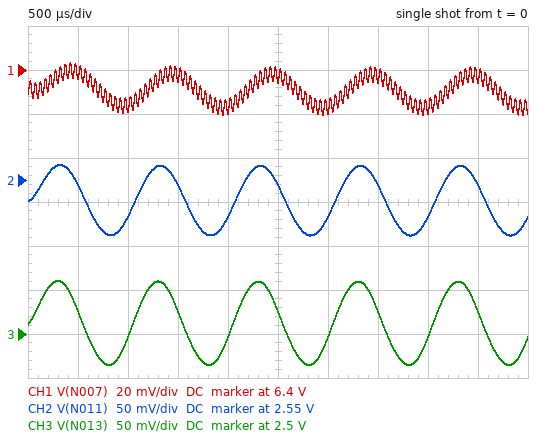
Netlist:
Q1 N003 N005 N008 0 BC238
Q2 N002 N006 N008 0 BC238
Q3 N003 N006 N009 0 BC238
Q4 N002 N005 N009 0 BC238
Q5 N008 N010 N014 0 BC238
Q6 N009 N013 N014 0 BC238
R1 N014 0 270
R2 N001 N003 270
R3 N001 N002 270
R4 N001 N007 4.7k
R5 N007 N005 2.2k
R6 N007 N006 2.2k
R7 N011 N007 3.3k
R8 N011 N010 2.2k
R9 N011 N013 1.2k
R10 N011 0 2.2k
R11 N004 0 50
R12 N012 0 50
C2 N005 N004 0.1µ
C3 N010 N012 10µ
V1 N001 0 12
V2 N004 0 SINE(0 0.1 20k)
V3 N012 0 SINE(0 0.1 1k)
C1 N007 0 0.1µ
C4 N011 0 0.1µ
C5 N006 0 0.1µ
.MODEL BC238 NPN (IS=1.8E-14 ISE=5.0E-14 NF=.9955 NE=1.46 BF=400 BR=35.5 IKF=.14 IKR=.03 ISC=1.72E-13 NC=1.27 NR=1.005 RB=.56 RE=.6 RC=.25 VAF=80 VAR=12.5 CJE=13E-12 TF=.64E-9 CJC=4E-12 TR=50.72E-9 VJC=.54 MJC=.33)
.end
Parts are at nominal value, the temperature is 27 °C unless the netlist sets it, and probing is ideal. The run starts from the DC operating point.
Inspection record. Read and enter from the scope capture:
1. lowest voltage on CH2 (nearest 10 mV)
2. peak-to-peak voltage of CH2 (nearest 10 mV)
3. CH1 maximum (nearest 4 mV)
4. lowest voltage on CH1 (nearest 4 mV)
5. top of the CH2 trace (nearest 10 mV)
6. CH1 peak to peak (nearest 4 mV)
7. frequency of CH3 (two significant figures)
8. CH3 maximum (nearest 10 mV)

2.49 V
80 mV
6.404 V
6.380 V
2.57 V
24 mV
1.0 kHz
2.56 V
